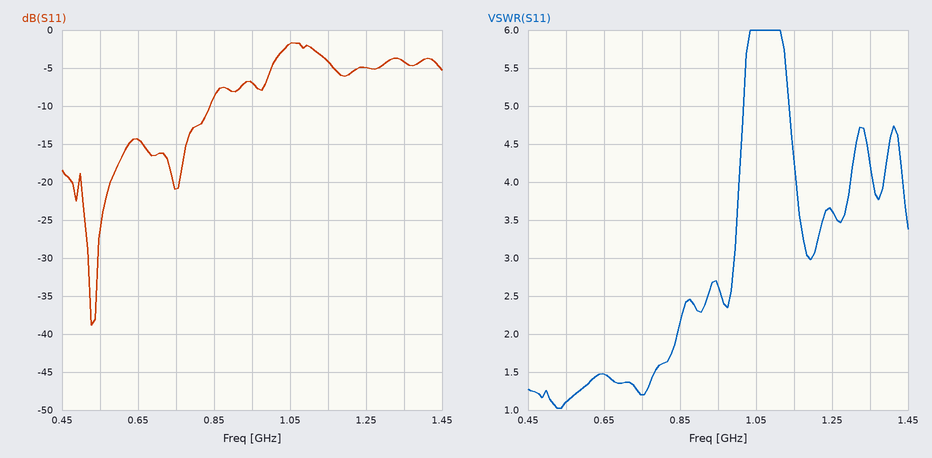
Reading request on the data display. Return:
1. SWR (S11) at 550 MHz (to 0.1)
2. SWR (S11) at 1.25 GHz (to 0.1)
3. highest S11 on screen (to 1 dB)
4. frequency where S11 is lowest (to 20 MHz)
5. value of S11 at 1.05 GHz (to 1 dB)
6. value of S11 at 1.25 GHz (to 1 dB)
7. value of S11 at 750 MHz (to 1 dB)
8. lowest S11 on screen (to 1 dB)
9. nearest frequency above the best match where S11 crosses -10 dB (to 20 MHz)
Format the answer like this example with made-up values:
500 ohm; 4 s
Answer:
1.1; 3.6; -2 dB; 520 MHz; -2 dB; -5 dB; -21 dB; -39 dB; 840 MHz
